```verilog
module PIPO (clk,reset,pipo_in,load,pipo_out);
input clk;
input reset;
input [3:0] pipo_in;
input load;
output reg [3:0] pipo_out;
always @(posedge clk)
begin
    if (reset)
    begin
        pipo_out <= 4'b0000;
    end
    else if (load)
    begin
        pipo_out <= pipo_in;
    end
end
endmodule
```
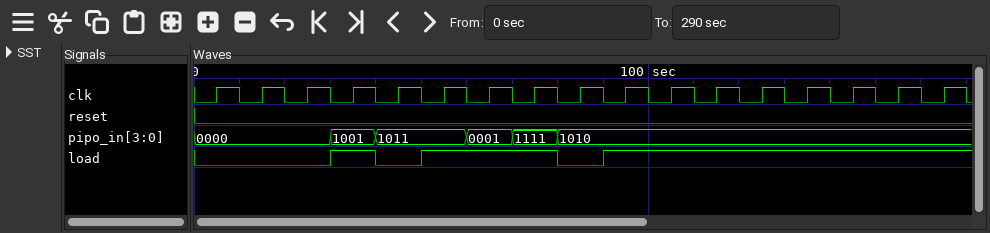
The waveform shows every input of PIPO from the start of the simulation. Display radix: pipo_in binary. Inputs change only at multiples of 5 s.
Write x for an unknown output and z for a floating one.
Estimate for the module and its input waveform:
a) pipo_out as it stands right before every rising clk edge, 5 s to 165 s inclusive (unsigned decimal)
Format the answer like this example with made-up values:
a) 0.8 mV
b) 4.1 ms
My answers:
a) x, x, x, x, 9, 9, 11, 1, 15, 15, 10, 10, 10, 10, 10, 10, 10
